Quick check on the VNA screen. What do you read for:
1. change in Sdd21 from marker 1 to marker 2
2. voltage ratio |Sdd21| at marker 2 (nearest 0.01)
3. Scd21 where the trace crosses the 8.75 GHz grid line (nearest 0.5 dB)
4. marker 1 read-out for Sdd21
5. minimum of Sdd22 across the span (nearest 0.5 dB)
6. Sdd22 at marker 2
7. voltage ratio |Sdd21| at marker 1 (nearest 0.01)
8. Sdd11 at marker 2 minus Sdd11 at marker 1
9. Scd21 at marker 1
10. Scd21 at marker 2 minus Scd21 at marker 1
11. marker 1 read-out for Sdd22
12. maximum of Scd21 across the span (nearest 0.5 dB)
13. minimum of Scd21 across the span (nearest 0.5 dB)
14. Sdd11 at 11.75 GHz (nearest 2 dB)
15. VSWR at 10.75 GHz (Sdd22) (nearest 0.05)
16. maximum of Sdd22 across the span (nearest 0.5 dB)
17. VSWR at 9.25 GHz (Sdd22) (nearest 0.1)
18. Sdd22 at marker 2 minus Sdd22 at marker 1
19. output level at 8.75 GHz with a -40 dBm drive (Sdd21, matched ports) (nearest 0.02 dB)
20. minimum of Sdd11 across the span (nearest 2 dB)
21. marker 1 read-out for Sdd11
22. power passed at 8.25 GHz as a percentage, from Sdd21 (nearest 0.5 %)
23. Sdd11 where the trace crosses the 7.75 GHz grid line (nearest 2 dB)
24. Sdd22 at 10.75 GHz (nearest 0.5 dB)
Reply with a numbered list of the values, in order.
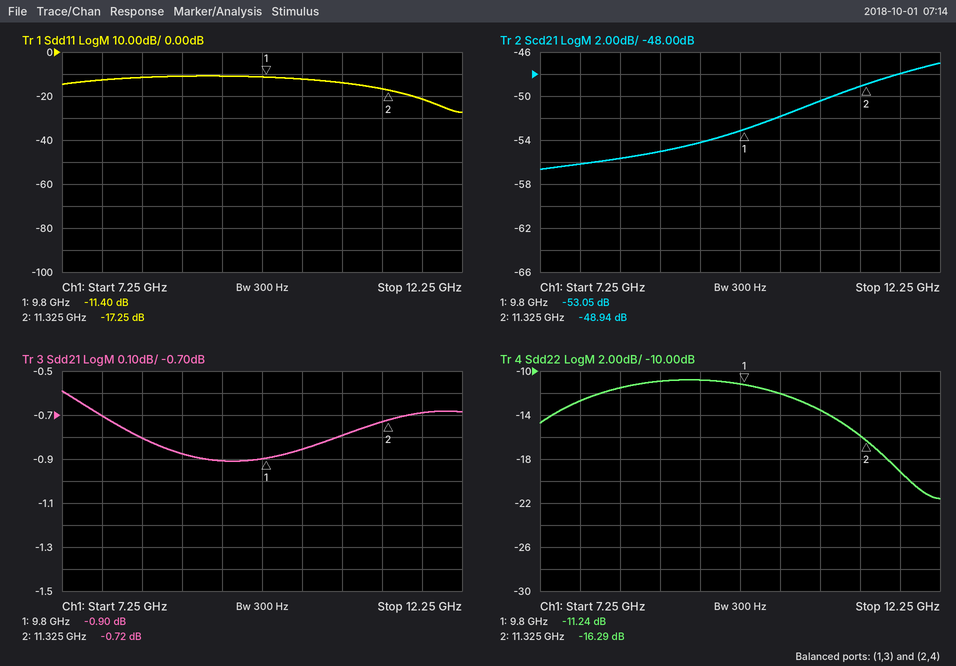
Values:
1. 0.18 dB
2. 0.92
3. -55.0 dB
4. -0.90 dB
5. -21.5 dB
6. -16.29 dB
7. 0.90
8. -5.85 dB
9. -53.05 dB
10. 4.11 dB
11. -11.24 dB
12. -47.0 dB
13. -56.5 dB
14. -22 dB
15. 1.55
16. -11.0 dB
17. 1.8
18. -5.05 dB
19. -40.88 dBm
20. -28 dB
21. -11.40 dB
22. 83.0 %
23. -12 dB
24. -13.5 dB
